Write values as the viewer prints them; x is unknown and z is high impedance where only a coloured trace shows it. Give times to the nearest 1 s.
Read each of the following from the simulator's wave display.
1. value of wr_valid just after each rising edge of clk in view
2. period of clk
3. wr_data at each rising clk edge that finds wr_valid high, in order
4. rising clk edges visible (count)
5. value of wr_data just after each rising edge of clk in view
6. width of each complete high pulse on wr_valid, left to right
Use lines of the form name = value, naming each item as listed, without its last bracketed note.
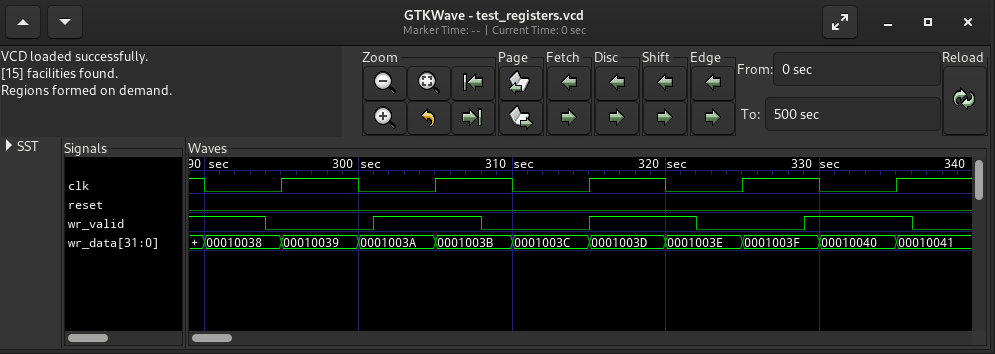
value of wr_valid just after each rising edge of clk in view = 0 1 1 0 1
period of clk = 10 s
wr_data at each rising clk edge that finds wr_valid high, in order = 0001003A, 00010040
rising clk edges visible = 5
value of wr_data just after each rising edge of clk in view = 00010039, 0001003B, 0001003D, 0001003F, 00010041
width of each complete high pulse on wr_valid, left to right = 7 s, 7 s, 7 s
